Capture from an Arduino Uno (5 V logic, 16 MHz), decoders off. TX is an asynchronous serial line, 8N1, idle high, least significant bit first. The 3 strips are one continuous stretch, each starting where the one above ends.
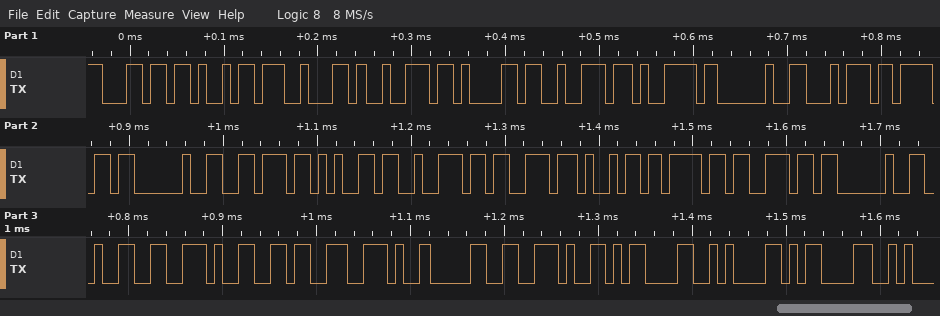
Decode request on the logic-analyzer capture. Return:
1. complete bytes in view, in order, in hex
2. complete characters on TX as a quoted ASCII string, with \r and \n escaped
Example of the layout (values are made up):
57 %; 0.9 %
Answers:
0x6C 0x69 0x62 0x72 0x61 0x72 0x79 0x20 0x74 0x6F 0x20 0x76 0x65 0x72 0x73 0x69 0x6F 0x6E 0x20 0x32 0x2E 0x36 0x2E 0x30 0x2E 0x0D 0x0A 0x0D; "library to version 2.6.0.\r\n\r"
